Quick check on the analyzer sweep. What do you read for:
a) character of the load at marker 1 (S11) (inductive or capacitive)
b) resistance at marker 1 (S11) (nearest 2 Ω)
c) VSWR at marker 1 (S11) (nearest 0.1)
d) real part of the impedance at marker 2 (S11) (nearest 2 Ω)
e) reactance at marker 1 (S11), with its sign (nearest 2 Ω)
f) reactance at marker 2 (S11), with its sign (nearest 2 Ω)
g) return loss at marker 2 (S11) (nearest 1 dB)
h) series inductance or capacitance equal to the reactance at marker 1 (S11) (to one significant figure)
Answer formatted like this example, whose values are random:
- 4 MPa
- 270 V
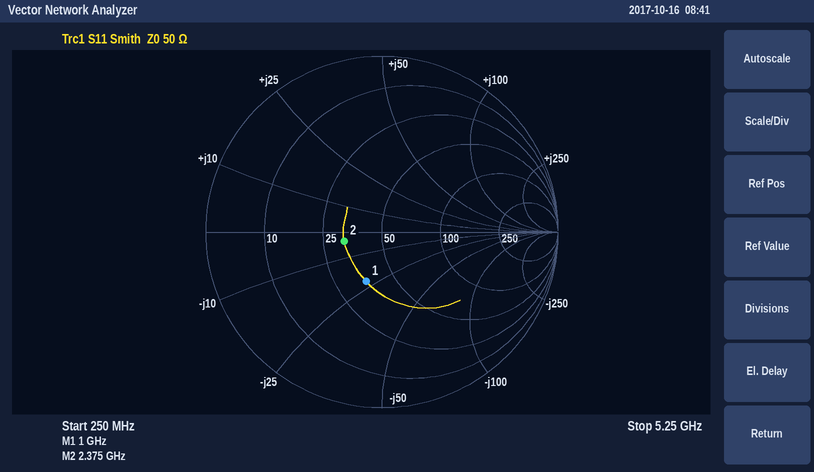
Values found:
- capacitive
- 36 Ω
- 1.8
- 32 Ω
- -22 Ω
- -4 Ω
- 13 dB
- 7 pF
